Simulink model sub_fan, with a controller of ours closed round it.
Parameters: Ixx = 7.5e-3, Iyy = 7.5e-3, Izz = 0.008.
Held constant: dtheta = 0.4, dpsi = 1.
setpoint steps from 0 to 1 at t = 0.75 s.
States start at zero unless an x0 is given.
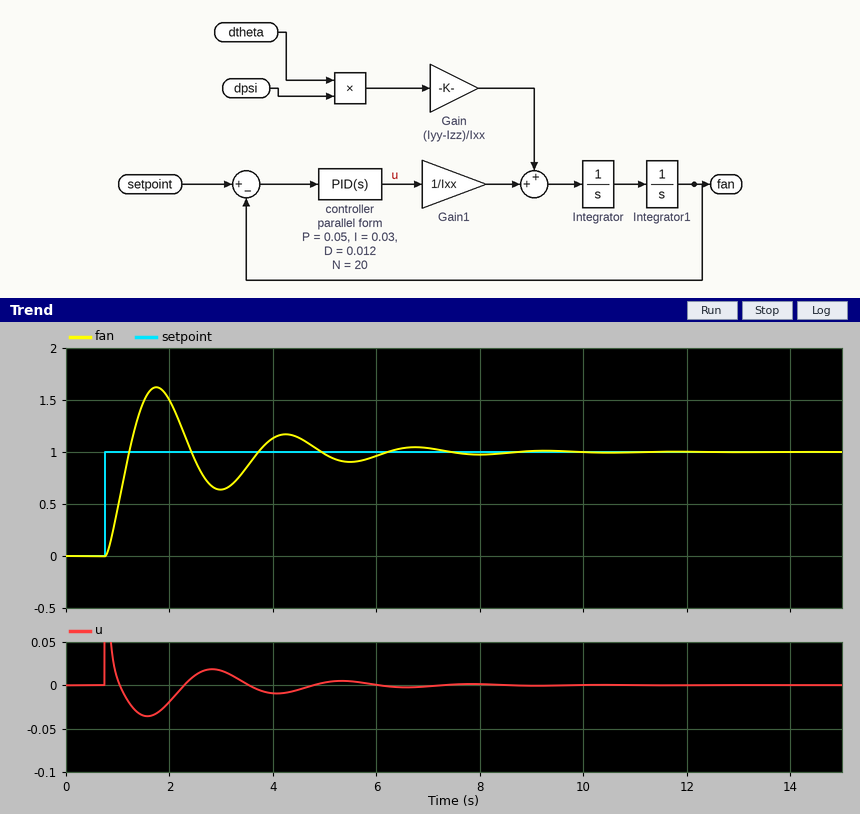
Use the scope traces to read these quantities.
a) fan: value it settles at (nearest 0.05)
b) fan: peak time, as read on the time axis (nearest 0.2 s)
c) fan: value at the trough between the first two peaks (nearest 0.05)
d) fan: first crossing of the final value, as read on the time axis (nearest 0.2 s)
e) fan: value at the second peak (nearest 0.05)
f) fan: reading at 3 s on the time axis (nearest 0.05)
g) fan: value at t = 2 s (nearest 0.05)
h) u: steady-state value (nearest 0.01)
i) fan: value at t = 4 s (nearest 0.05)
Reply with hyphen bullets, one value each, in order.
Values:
- 1.00
- 1.8 s
- 0.65
- 1.2 s
- 1.15
- 0.65
- 1.50
- 0.00
- 1.15
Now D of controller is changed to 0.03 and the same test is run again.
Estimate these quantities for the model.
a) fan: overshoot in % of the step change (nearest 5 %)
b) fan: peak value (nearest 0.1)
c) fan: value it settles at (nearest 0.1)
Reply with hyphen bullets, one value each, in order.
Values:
- 25 %
- 1.3
- 1.0
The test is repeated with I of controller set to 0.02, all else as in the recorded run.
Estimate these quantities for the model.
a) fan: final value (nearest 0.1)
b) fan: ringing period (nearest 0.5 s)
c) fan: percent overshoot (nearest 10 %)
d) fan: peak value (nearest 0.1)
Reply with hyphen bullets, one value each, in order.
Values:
- 1.0
- 2.5 s
- 60 %
- 1.6
